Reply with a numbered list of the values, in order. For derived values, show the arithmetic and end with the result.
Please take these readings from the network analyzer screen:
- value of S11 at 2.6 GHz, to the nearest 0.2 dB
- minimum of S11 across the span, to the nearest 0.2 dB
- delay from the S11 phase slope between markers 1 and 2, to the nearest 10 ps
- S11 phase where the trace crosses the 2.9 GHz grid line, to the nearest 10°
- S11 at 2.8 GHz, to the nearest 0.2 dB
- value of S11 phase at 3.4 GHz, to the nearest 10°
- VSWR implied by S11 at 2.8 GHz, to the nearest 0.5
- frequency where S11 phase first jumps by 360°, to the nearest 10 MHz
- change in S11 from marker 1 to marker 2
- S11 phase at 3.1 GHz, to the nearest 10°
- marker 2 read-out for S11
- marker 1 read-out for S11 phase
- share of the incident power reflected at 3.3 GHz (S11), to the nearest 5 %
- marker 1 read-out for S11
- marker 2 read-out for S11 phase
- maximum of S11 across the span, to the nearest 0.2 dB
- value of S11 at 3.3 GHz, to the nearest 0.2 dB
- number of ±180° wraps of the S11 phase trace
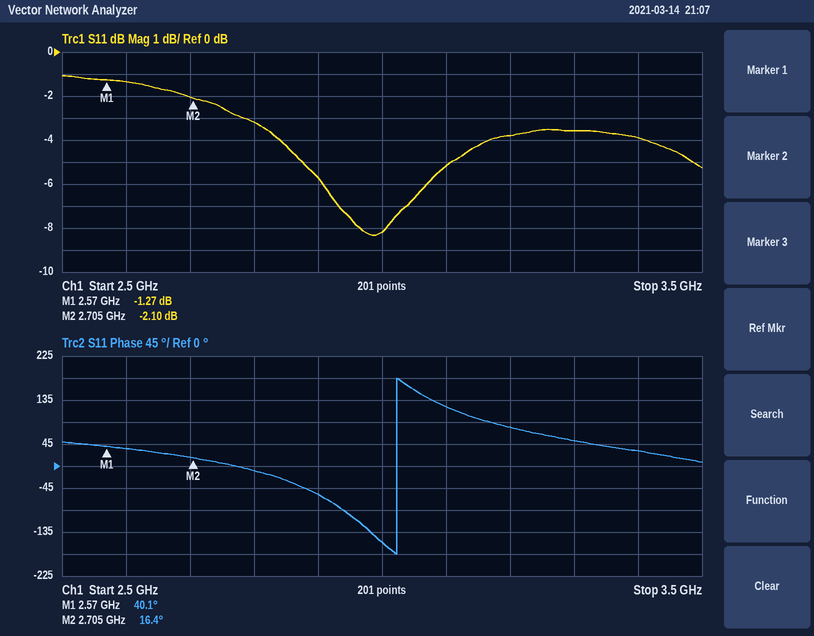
1. -1.4 dB
2. -8.4 dB
3. −(16.4° − (40.1°))/(360° × 135 MHz) ≈ 488 ps, so 490 ps to the nearest 10 ps
4. -60°
5. -3.2 dB
6. 30°
7. |Γ| = 10^(-3.2/20) = 0.6918; VSWR = (1 + 0.6918)/(1 − 0.6918) ≈ 5.5
8. 3.02 GHz
9. -2.1 − (-1.27) = -0.83 dB
10. 120°
11. -2.10 dB
12. 40.1°
13. 10^(-3.6/10) ≈ 43.7 %, so 45 % to the nearest 5 %
14. -1.27 dB
15. 16.4°
16. -1.0 dB
17. -3.6 dB
18. 1
